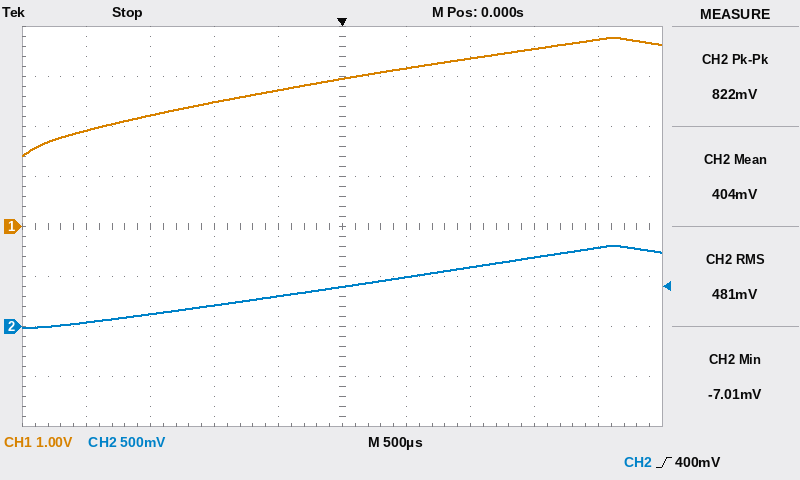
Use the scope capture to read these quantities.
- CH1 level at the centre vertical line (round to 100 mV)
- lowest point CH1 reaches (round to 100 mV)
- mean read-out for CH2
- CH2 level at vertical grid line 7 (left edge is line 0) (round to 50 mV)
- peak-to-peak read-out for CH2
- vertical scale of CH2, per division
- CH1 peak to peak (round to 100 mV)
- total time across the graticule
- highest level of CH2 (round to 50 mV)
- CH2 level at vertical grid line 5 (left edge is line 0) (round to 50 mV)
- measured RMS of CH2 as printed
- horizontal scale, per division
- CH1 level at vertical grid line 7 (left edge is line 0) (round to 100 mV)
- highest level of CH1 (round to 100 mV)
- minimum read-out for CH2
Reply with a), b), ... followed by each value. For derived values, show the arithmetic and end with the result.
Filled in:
a) 3.0 V
b) 1.4 V
c) 404 mV
d) 600 mV
e) 822 mV
f) 500 mV
g) 3.8 V − (1.4 V) = 2.4 V
h) 5 ms
i) 800 mV
j) 400 mV
k) 481 mV
l) 500 µs
m) 3.4 V
n) 3.8 V
o) -7.01 mV
